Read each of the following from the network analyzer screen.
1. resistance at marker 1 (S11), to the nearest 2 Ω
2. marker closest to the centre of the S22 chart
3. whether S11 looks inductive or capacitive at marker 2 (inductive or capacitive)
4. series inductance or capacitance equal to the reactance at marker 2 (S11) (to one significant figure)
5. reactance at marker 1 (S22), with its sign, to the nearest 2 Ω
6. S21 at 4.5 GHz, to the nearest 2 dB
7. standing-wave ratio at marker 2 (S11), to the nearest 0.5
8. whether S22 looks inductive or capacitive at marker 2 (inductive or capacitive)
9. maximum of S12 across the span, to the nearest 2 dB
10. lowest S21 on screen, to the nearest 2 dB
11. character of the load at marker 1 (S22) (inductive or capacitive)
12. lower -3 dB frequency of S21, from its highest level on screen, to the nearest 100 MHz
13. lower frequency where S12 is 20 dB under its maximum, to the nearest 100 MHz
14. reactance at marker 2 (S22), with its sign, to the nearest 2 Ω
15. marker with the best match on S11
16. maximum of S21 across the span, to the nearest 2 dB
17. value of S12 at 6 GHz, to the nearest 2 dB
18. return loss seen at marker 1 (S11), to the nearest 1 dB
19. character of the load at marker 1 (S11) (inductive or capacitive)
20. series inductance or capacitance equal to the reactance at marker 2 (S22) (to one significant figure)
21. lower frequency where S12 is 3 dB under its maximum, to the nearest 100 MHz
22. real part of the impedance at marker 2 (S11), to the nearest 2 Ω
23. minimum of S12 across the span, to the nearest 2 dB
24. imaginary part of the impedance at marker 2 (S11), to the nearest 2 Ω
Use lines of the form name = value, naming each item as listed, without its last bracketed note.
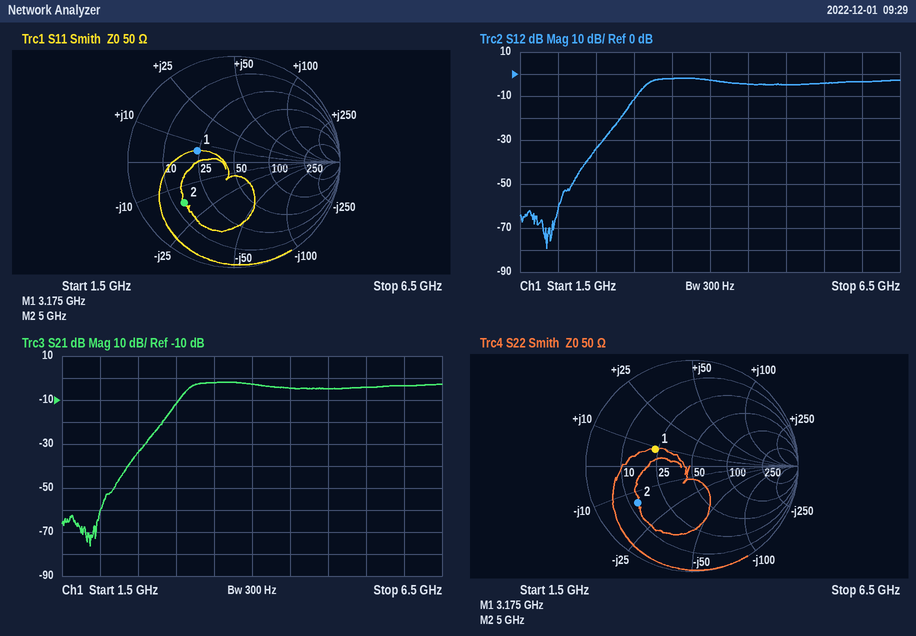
resistance at marker 1 (S11), to the nearest 2 Ω = 24 Ω
marker closest to the centre of the S22 chart = marker 1
whether S11 looks inductive or capacitive at marker 2 = capacitive
series inductance or capacitance equal to the reactance at marker 2 (S11) = 2 pF
reactance at marker 1 (S22), with its sign, to the nearest 2 Ω = +8 Ω
S21 at 4.5 GHz, to the nearest 2 dB = -4 dB
standing-wave ratio at marker 2 (S11), to the nearest 0.5 = 4.0
whether S22 looks inductive or capacitive at marker 2 = capacitive
maximum of S12 across the span, to the nearest 2 dB = -2 dB
lowest S21 on screen, to the nearest 2 dB = -76 dB
character of the load at marker 1 (S22) = inductive
lower -3 dB frequency of S21, from its highest level on screen, to the nearest 100 MHz = 3.2 GHz
lower frequency where S12 is 20 dB under its maximum, to the nearest 100 MHz = 2.8 GHz
reactance at marker 2 (S22), with its sign, to the nearest 2 Ω = -14 Ω
marker with the best match on S11 = marker 1
maximum of S21 across the span, to the nearest 2 dB = -2 dB
value of S12 at 6 GHz, to the nearest 2 dB = -4 dB
return loss seen at marker 1 (S11), to the nearest 1 dB = 9 dB
character of the load at marker 1 (S11) = inductive
series inductance or capacitance equal to the reactance at marker 2 (S22) = 2 pF
lower frequency where S12 is 3 dB under its maximum, to the nearest 100 MHz = 3.2 GHz
real part of the impedance at marker 2 (S11), to the nearest 2 Ω = 14 Ω
minimum of S12 across the span, to the nearest 2 dB = -80 dB
imaginary part of the impedance at marker 2 (S11), to the nearest 2 Ω = -16 Ω
